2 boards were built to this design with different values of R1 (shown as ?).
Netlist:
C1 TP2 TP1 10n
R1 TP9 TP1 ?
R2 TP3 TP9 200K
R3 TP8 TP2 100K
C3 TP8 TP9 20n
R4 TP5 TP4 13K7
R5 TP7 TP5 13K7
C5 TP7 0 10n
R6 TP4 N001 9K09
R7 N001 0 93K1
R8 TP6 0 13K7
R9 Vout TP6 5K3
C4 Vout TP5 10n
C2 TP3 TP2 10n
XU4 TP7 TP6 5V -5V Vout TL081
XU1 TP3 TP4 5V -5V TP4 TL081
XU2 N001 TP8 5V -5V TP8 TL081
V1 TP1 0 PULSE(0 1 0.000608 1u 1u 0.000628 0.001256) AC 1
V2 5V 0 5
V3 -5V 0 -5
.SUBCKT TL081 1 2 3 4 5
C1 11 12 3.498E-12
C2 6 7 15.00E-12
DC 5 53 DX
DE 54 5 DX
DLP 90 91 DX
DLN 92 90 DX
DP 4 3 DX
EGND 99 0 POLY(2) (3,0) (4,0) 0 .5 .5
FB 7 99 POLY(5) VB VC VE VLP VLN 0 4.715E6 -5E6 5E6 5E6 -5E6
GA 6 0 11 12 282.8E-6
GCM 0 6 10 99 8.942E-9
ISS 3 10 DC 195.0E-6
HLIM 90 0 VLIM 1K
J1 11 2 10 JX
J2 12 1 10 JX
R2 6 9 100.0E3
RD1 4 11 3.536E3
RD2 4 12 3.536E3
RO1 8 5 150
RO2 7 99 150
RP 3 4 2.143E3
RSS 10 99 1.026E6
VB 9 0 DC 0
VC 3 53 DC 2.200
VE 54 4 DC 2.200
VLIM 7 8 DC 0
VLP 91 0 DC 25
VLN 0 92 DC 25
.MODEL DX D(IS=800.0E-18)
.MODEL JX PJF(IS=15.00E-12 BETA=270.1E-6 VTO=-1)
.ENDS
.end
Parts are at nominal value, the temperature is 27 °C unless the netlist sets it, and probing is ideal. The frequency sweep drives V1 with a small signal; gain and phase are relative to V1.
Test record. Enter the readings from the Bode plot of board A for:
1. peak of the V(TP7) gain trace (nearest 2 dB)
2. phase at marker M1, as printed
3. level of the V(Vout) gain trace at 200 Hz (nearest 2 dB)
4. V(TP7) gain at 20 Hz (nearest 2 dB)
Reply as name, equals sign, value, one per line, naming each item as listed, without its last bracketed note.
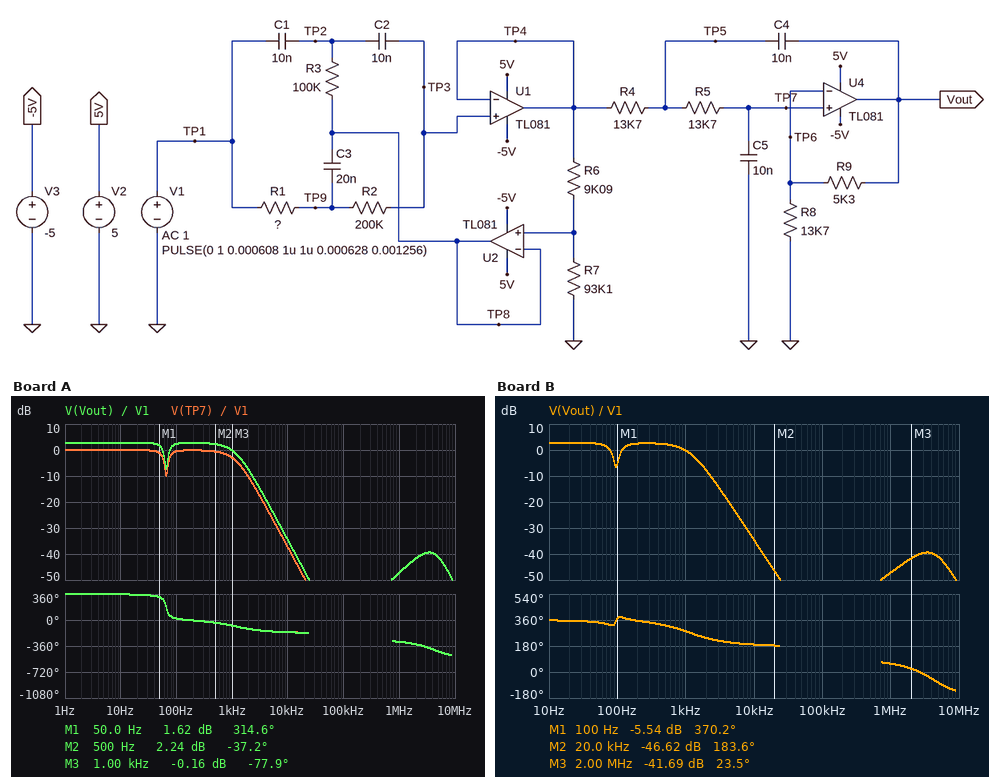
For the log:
peak of the V(TP7) gain trace = 0 dB
phase at marker M1, as printed = 314.6 deg
level of the V(Vout) gain trace at 200 Hz = 2 dB
V(TP7) gain at 20 Hz = 0 dB
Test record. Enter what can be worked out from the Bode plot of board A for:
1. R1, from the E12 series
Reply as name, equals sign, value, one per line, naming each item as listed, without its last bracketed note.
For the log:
R1, from the E12 series = 330 kΩ
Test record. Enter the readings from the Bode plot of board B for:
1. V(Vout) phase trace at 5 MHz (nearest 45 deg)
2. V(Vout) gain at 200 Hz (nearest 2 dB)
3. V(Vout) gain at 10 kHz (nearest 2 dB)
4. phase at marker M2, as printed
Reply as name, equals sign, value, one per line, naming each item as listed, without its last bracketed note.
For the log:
V(Vout) phase trace at 5 MHz = -90 deg
V(Vout) gain at 200 Hz = 2 dB
V(Vout) gain at 10 kHz = -34 dB
phase at marker M2, as printed = 183.6 deg
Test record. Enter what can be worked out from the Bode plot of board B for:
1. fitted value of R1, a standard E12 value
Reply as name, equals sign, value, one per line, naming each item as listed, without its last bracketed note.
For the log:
fitted value of R1, a standard E12 value = 120 kΩ
